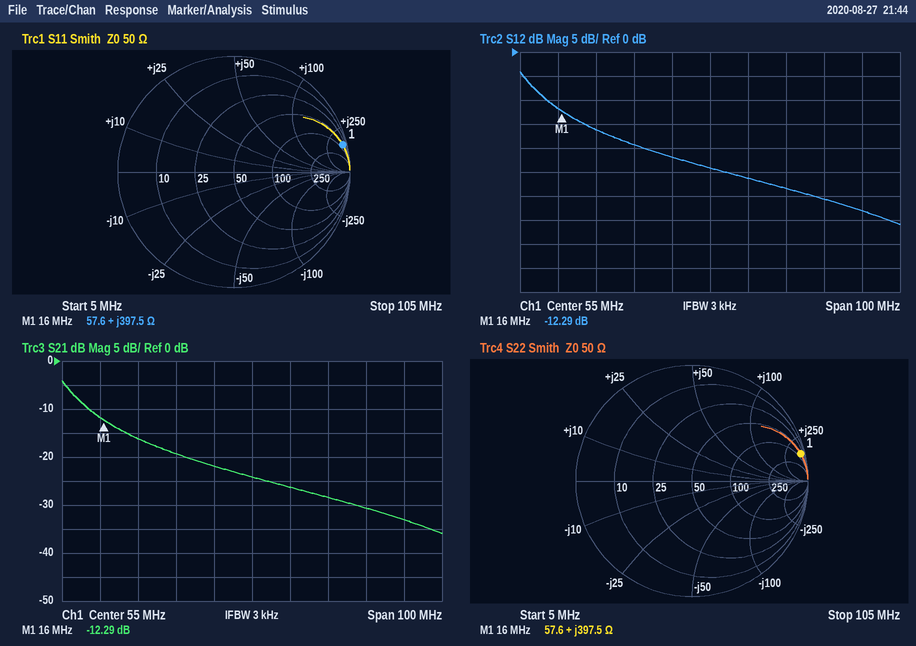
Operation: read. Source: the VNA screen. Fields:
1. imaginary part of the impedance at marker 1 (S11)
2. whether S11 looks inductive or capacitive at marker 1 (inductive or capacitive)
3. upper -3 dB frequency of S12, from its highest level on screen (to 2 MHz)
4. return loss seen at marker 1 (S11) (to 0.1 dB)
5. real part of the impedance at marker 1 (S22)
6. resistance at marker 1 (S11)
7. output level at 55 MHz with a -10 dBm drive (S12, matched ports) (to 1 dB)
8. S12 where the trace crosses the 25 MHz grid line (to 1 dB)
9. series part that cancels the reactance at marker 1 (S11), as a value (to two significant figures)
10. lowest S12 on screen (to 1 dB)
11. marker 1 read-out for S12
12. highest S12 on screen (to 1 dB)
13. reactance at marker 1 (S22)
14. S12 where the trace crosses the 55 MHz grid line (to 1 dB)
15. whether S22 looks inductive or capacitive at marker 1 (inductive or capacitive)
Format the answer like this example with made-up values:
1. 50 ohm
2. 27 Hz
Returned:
1. +397.5 Ω
2. inductive
3. 8 MHz
4. 0.3 dB
5. 57.6 Ω
6. 57.6 Ω
7. -34 dBm
8. -16 dB
9. 25 pF
10. -36 dB
11. -12.29 dB
12. -4 dB
13. +397.5 Ω
14. -24 dB
15. inductive
